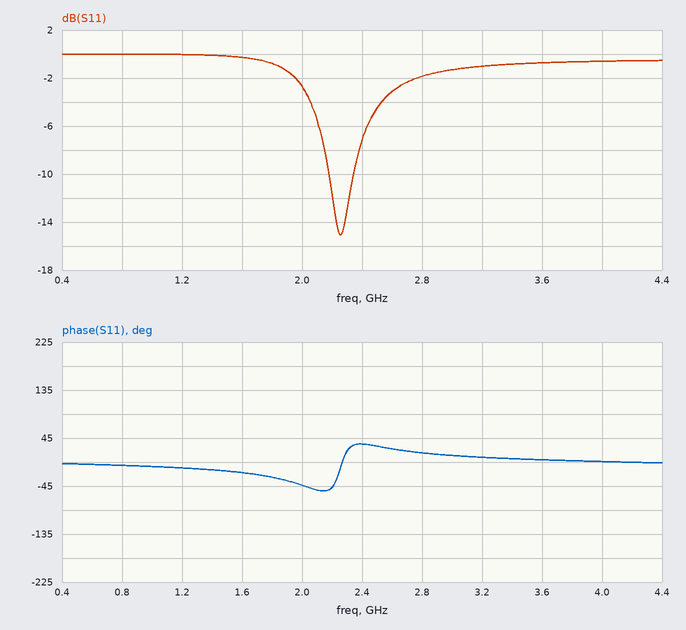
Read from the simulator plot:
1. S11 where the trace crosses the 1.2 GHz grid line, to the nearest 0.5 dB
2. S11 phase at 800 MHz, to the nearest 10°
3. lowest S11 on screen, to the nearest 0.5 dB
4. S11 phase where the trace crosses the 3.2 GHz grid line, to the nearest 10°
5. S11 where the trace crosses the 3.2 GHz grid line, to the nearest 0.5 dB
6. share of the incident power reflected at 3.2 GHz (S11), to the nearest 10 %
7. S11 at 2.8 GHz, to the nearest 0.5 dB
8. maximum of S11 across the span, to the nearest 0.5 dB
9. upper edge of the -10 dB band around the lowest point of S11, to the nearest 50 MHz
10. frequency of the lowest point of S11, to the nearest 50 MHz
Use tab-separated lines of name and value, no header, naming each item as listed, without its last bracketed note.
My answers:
S11 where the trace crosses the 1.2 GHz grid line, to the nearest 0.5 dB	0.0 dB
S11 phase at 800 MHz, to the nearest 10°	-10°
lowest S11 on screen, to the nearest 0.5 dB	-15.0 dB
S11 phase where the trace crosses the 3.2 GHz grid line, to the nearest 10°	10°
S11 where the trace crosses the 3.2 GHz grid line, to the nearest 0.5 dB	-1.0 dB
share of the incident power reflected at 3.2 GHz (S11), to the nearest 10 %	80 %
S11 at 2.8 GHz, to the nearest 0.5 dB	-2.0 dB
maximum of S11 across the span, to the nearest 0.5 dB	0.0 dB
upper edge of the -10 dB band around the lowest point of S11, to the nearest 50 MHz	2.35 GHz
frequency of the lowest point of S11, to the nearest 50 MHz	2.25 GHz
